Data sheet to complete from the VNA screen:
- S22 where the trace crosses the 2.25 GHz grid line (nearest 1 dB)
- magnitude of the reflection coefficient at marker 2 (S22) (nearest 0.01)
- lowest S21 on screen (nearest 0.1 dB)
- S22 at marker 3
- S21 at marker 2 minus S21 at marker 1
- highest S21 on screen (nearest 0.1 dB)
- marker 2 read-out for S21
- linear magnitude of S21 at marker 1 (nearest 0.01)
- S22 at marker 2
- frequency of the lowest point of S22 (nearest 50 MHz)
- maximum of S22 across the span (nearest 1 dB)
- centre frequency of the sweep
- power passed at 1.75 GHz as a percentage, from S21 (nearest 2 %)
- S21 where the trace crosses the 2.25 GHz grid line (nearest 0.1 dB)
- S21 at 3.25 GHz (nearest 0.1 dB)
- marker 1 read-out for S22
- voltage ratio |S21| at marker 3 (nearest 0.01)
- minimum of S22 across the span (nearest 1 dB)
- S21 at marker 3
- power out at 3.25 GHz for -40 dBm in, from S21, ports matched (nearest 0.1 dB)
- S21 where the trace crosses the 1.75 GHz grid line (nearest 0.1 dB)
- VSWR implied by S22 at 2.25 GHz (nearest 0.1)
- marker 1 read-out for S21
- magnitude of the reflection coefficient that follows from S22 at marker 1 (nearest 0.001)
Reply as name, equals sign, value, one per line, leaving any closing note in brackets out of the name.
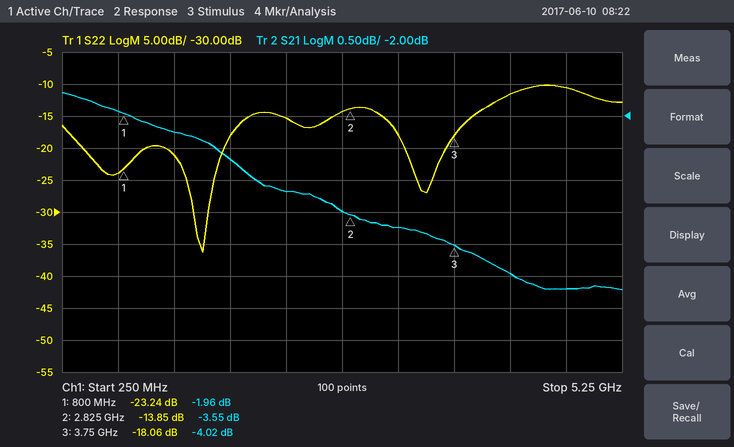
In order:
S22 where the trace crosses the 2.25 GHz grid line = -15 dB
magnitude of the reflection coefficient at marker 2 (S22) = 0.20
lowest S21 on screen = -4.7 dB
S22 at marker 3 = -18.06 dB
S21 at marker 2 minus S21 at marker 1 = -1.59 dB
highest S21 on screen = -1.6 dB
marker 2 read-out for S21 = -3.55 dB
linear magnitude of S21 at marker 1 = 0.80
S22 at marker 2 = -13.85 dB
frequency of the lowest point of S22 = 1.50 GHz
maximum of S22 across the span = -10 dB
centre frequency of the sweep = 2.75 GHz
power passed at 1.75 GHz as a percentage, from S21 = 54 %
S21 where the trace crosses the 2.25 GHz grid line = -3.2 dB
S21 at 3.25 GHz = -3.7 dB
marker 1 read-out for S22 = -23.24 dB
voltage ratio |S21| at marker 3 = 0.63
minimum of S22 across the span = -36 dB
S21 at marker 3 = -4.02 dB
power out at 3.25 GHz for -40 dBm in, from S21, ports matched = -43.7 dBm
S21 where the trace crosses the 1.75 GHz grid line = -2.7 dB
VSWR implied by S22 at 2.25 GHz = 1.4
marker 1 read-out for S21 = -1.96 dB
magnitude of the reflection coefficient that follows from S22 at marker 1 = 0.069
